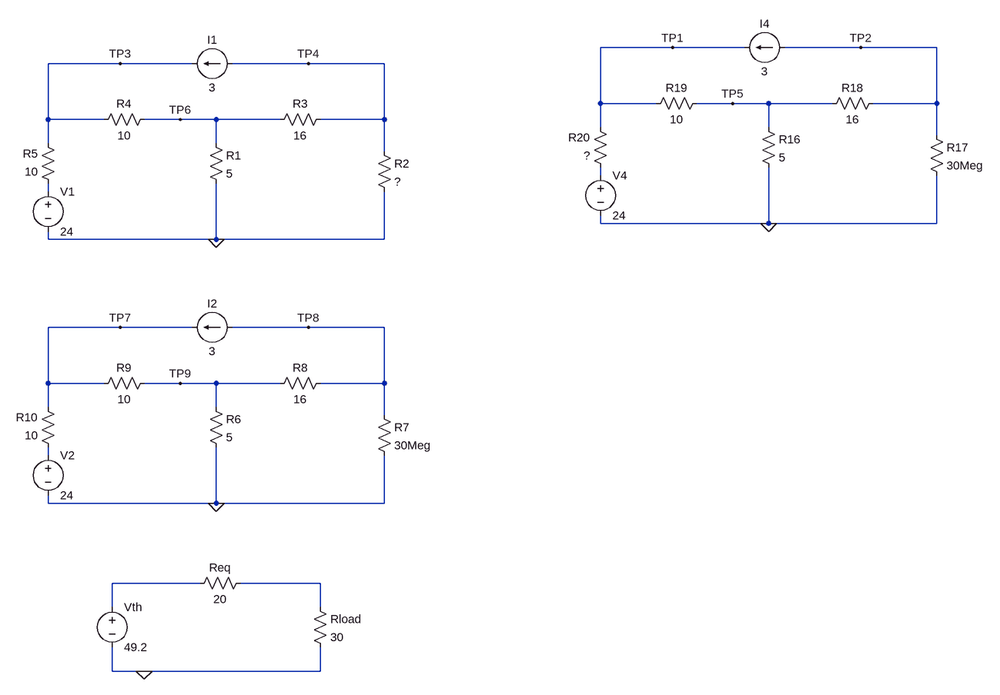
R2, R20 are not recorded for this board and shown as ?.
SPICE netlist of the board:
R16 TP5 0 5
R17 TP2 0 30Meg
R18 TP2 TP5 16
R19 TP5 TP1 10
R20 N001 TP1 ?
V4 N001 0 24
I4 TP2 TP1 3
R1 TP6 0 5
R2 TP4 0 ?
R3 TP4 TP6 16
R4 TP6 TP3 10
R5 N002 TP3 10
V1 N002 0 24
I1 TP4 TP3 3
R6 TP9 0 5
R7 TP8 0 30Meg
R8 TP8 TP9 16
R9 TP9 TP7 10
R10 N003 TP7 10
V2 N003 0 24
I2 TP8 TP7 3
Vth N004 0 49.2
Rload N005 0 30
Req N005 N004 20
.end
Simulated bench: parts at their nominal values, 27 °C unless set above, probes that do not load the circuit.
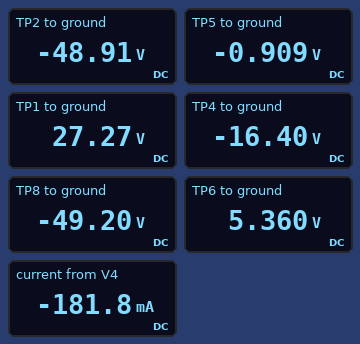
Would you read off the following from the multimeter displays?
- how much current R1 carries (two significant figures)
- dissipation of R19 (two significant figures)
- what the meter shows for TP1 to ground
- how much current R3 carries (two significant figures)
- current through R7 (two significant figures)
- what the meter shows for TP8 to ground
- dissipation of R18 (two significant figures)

1.1 A
79 W
27.27 V
1.4 A
1.6 µA
-49.20 V
140 W
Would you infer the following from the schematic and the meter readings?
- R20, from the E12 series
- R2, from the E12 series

18 Ω
10 Ω
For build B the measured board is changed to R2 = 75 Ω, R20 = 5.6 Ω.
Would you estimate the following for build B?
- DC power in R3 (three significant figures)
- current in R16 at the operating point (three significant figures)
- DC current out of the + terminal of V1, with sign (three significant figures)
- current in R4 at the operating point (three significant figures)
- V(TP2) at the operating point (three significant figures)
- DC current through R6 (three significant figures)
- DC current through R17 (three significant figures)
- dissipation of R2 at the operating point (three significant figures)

98.6 W
291 mA
-344 mA
2.66 A
-49.5 V
240 mA
1.65 µA
20.1 W
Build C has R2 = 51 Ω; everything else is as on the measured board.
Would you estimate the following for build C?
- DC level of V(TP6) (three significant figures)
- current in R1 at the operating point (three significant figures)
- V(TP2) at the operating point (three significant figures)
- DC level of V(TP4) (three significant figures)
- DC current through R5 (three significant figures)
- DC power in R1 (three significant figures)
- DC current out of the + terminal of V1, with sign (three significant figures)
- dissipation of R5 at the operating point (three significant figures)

1.57 V
314 mA
-48.9 V
-35.3 V
379 mA
494 mW
-379 mA
1.43 W
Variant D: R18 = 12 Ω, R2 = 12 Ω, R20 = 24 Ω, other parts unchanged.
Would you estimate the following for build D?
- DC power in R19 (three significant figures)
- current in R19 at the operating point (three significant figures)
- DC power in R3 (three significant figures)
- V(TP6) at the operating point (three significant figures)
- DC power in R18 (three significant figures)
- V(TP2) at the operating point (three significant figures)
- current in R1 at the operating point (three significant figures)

81.0 W
2.85 A
34.2 W
4.95 V
108 W
-36.8 V
990 mA
